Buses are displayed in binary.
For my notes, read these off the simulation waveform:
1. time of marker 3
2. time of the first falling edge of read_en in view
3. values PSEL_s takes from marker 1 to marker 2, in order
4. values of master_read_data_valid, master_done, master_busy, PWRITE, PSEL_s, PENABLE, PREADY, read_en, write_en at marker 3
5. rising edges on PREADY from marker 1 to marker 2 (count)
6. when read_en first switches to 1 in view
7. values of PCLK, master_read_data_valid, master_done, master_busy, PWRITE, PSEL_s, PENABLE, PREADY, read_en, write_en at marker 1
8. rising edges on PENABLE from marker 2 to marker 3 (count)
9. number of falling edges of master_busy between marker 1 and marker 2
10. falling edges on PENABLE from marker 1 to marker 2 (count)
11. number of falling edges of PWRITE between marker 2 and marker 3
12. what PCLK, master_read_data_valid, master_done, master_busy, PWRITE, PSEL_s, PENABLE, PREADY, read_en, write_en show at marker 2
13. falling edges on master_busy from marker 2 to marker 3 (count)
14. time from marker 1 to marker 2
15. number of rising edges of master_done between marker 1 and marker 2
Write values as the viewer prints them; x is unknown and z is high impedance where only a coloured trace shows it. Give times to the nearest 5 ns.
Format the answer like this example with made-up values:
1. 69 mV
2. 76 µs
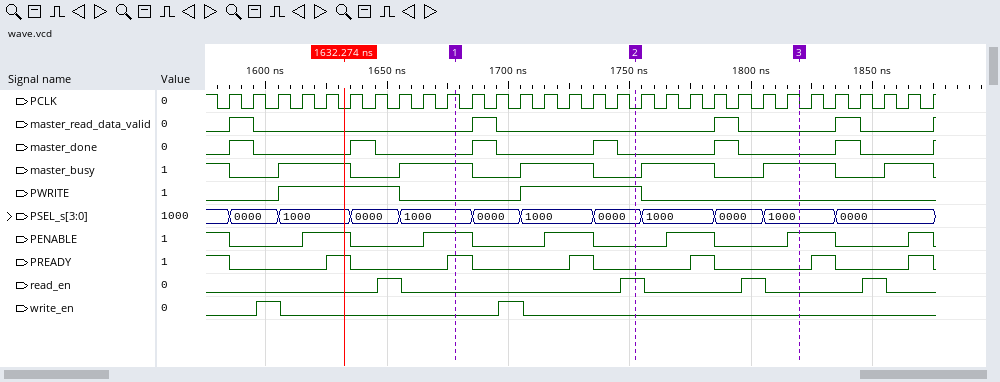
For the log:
1. 1820 ns
2. 1655 ns
3. 1000, 0000, 1000, 0000
4. master_read_data_valid=0, master_done=0, master_busy=1, PWRITE=0, PSEL_s=1000, PENABLE=1, PREADY=0, read_en=0, write_en=0
5. 1
6. 1645 ns
7. PCLK=1, master_read_data_valid=0, master_done=0, master_busy=1, PWRITE=0, PSEL_s=1000, PENABLE=1, PREADY=1, read_en=0, write_en=0
8. 2
9. 2
10. 2
11. 1
12. PCLK=0, master_read_data_valid=0, master_done=0, master_busy=0, PWRITE=1, PSEL_s=0000, PENABLE=0, PREADY=0, read_en=1, write_en=0
13. 1
14. 75 ns
15. 2
